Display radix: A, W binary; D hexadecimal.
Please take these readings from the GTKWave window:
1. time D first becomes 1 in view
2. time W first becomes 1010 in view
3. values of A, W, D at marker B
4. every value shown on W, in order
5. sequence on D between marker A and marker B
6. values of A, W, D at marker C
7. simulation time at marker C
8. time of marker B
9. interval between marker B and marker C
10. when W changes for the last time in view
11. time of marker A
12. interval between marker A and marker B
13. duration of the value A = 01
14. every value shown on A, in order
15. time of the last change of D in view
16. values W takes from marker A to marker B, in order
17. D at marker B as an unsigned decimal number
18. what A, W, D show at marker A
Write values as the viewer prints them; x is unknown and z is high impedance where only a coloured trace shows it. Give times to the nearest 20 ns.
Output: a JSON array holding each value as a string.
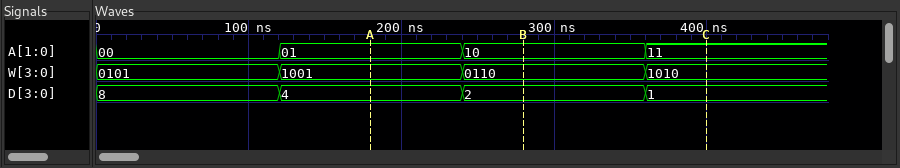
["360 ns", "360 ns", "A=10, W=0110, D=2", "0101, 1001, 0110, 1010", "4, 2", "A=11, W=1010, D=1", "400 ns", "280 ns", "120 ns", "360 ns", "180 ns", "100 ns", "120 ns", "00, 01, 10, 11", "360 ns", "1001, 0110", "2", "A=01, W=1001, D=4"]
